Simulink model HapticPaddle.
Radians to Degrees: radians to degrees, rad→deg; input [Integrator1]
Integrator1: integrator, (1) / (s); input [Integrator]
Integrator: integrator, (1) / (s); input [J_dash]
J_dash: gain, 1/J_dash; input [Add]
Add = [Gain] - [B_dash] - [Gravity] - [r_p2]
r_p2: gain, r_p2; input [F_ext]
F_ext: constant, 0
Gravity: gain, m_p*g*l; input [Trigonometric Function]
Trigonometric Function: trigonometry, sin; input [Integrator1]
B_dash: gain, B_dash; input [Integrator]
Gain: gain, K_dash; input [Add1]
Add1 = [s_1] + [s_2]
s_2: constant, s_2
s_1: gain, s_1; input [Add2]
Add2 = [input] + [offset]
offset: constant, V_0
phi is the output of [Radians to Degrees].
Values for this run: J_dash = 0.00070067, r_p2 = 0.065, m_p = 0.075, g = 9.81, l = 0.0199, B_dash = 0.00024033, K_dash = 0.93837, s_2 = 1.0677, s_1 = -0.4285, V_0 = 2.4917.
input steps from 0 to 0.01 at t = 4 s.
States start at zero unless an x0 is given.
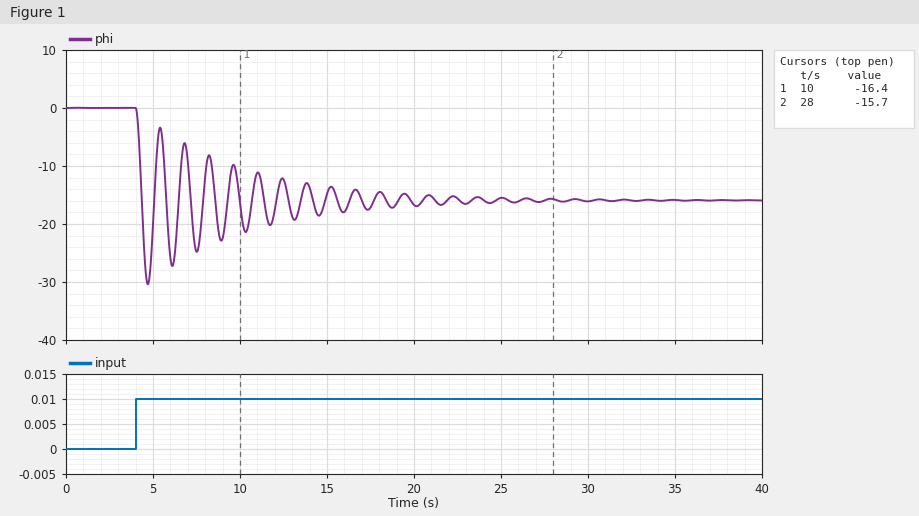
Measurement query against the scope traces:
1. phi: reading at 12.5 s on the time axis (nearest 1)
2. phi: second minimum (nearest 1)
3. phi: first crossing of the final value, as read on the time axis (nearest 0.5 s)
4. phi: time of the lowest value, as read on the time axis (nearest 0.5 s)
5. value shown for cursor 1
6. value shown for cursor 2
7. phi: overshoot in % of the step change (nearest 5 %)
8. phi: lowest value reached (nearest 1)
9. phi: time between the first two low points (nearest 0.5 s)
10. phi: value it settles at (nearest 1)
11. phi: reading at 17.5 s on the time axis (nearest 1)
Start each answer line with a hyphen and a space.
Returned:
- -12
- -27
- 4.5 s
- 4.5 s
- -16.4
- -15.7
- 90 %
- -30
- 1.5 s
- -16
- -17
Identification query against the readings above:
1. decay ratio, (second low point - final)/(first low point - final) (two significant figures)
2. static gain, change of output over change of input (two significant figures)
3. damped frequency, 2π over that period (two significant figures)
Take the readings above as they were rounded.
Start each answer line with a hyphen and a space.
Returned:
- 0.79
- -1600
- 4.2 rad/s
